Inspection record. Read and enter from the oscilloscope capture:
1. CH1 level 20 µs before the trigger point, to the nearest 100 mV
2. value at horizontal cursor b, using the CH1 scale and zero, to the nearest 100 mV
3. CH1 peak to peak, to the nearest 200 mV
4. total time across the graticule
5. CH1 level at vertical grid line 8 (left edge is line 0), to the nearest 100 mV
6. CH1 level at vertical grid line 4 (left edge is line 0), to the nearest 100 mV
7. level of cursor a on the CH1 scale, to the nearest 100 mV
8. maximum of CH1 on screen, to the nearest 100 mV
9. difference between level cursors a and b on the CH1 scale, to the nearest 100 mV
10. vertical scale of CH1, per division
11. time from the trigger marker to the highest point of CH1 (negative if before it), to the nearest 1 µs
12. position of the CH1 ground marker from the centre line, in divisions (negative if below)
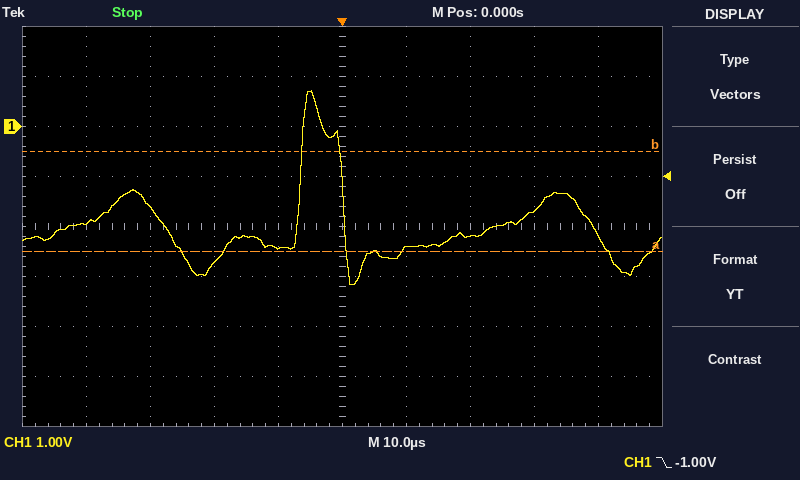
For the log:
-2.7 V
-500 mV
3.8 V
100 µs
-1.7 V
-2.4 V
-2.5 V
700 mV
2.0 V
1 V
-5 µs
+2.0 div
